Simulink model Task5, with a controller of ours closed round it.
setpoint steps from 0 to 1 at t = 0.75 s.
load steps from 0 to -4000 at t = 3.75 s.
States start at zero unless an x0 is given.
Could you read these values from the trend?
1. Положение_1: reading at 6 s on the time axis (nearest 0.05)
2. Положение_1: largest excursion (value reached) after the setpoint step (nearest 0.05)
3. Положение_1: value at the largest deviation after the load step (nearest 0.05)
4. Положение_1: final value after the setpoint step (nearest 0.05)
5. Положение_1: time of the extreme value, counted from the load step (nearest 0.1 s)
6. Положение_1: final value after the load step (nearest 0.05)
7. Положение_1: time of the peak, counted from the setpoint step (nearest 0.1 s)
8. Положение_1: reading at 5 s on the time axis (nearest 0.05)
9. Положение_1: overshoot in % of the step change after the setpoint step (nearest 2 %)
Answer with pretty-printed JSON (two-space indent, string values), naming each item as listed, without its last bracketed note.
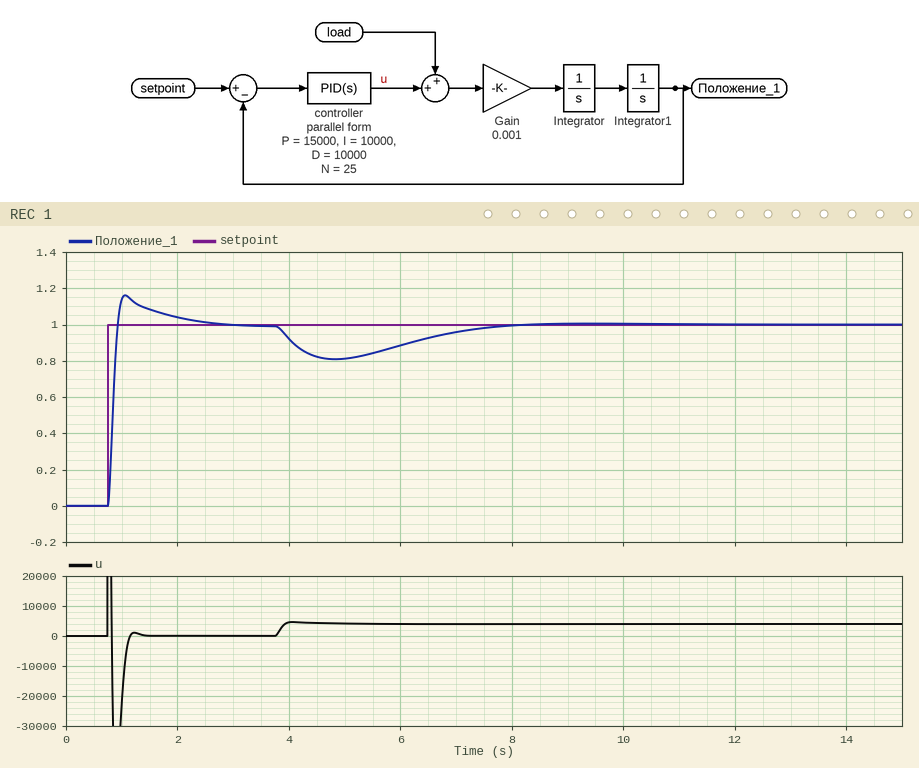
{
  "Положение_1: reading at 6 s on the time axis": "0.90",
  "Положение_1: largest excursion (value reached) after the setpoint step": "1.15",
  "Положение_1: value at the largest deviation after the load step": "0.80",
  "Положение_1: final value after the setpoint step": "1.00",
  "Положение_1: time of the extreme value, counted from the load step": "1.1 s",
  "Положение_1: final value after the load step": "1.00",
  "Положение_1: time of the peak, counted from the setpoint step": "0.3 s",
  "Положение_1: reading at 5 s on the time axis": "0.80",
  "Положение_1: overshoot in % of the step change after the setpoint step": "16 %"
}
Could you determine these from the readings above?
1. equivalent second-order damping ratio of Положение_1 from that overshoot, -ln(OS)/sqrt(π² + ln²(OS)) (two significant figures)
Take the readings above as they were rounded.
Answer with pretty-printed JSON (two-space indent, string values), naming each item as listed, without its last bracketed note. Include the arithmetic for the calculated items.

{
  "equivalent second-order damping ratio of Положение_1 from that overshoot, -ln(OS)/sqrt(π² + ln²(OS))": "ln(0.16) = -1.833; 1.833 / sqrt(9.870 + 3.358) = 0.50"
}
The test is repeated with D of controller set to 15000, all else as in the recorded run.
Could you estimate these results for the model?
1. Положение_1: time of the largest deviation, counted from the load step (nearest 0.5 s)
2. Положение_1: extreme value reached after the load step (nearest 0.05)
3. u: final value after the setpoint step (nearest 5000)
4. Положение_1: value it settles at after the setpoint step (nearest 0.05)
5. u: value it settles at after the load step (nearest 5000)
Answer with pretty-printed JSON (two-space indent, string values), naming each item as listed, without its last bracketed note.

{
  "Положение_1: time of the largest deviation, counted from the load step": "1.5 s",
  "Положение_1: extreme value reached after the load step": "0.85",
  "u: final value after the setpoint step": "0",
  "Положение_1: value it settles at after the setpoint step": "1.00",
  "u: value it settles at after the load step": "5000"
}
